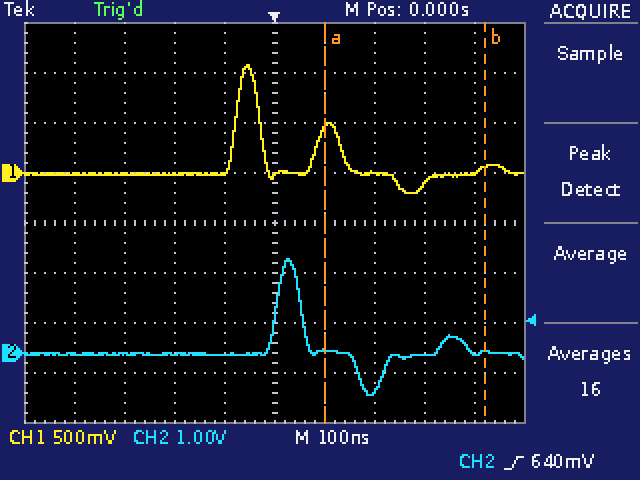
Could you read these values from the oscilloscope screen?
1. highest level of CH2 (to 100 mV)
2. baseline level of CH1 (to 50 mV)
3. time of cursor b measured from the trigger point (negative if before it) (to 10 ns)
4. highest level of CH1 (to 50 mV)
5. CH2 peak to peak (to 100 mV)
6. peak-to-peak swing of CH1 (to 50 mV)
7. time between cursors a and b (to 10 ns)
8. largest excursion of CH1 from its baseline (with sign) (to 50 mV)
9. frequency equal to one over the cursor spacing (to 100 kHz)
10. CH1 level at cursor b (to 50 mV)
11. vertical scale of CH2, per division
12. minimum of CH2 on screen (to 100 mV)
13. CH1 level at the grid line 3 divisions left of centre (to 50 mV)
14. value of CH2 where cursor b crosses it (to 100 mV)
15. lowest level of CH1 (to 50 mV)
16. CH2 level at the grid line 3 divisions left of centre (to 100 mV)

1.9 V
0 mV
+420 ns
1.10 V
2.7 V
1.30 V
320 ns
+1.10 V
3.1 MHz
50 mV
1 V
-800 mV
0 mV
0.0 V
-200 mV
0.0 V
